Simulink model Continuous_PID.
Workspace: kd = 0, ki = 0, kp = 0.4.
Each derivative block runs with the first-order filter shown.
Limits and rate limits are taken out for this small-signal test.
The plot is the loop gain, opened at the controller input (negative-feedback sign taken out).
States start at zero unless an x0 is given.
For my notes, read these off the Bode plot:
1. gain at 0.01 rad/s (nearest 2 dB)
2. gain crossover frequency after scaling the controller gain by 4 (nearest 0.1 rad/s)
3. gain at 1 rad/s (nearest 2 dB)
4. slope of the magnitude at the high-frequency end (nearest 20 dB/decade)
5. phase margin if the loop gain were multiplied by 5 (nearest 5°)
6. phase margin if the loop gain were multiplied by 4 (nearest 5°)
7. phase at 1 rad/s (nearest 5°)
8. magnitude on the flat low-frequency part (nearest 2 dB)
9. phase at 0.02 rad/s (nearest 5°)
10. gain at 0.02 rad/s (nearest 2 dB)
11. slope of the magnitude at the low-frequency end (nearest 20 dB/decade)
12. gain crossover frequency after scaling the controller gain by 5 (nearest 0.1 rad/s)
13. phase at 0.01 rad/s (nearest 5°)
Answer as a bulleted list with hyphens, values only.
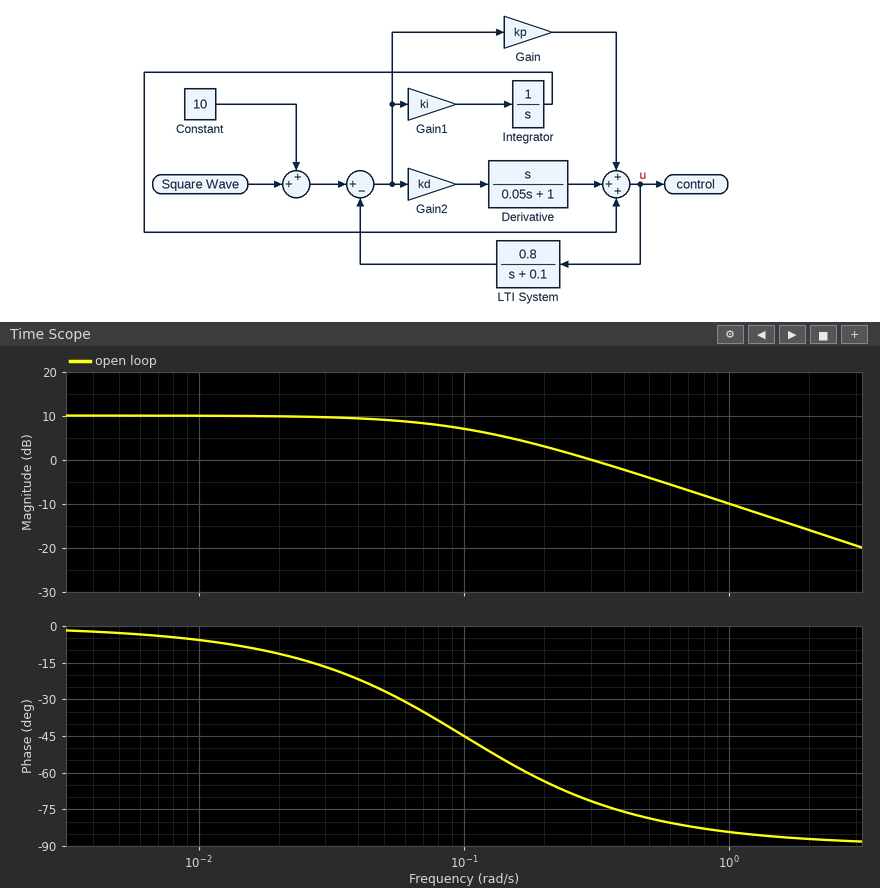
- 10 dB
- 1.3 rad/s
- -10 dB
- -20 dB/decade
- 95°
- 95°
- -85°
- 10 dB
- -10°
- 10 dB
- 0 dB/decade
- 1.6 rad/s
- -5°
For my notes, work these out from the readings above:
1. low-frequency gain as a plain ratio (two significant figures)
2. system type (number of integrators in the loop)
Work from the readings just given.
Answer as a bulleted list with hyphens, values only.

- 3.2
- 0
